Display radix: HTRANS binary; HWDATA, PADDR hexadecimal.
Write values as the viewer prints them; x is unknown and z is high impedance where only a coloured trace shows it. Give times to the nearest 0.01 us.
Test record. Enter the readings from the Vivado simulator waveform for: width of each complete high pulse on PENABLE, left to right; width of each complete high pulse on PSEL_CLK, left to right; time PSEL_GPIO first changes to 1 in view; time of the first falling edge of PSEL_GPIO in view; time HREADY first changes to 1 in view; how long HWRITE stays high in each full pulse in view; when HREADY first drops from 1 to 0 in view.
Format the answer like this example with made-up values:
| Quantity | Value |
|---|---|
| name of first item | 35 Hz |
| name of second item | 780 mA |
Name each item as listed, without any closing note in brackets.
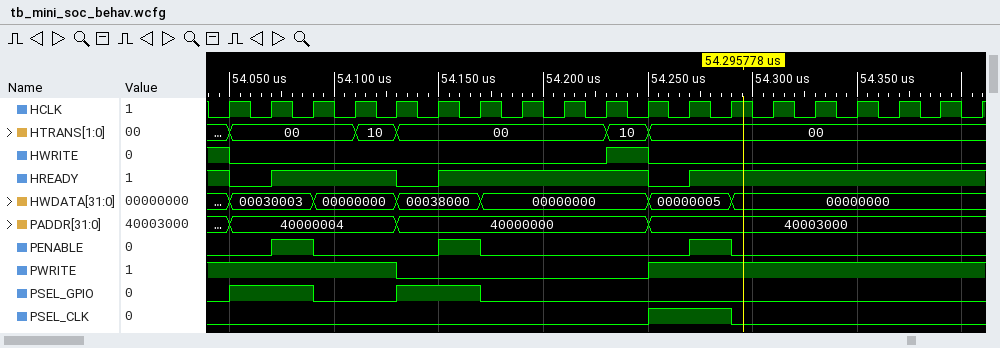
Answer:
| Quantity | Value |
|---|---|
| width of each complete high pulse on PENABLE, left to right | 0.02 us, 0.02 us, 0.02 us |
| width of each complete high pulse on PSEL_CLK, left to right | 0.04 us |
| time PSEL_GPIO first changes to 1 in view | 54.05 us |
| time of the first falling edge of PSEL_GPIO in view | 54.09 us |
| time HREADY first changes to 1 in view | 54.07 us |
| how long HWRITE stays high in each full pulse in view | 0.02 us |
| when HREADY first drops from 1 to 0 in view | 54.05 us |
